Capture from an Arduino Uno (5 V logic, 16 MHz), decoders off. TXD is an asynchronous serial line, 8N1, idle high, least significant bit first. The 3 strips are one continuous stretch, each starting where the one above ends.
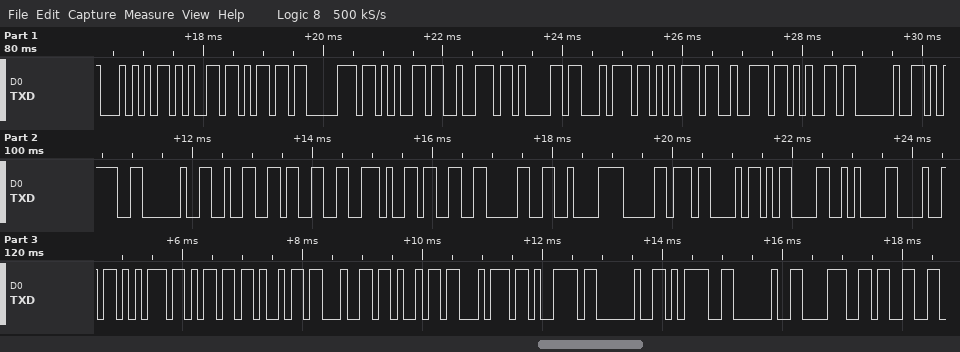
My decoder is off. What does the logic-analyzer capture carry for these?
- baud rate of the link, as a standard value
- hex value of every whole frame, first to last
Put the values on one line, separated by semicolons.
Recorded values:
9600 baud; 0x54 0x65 0x6D 0x70 0x65 0x72 0x61 0x74 0x75 0x72 0x65 0x20 0x3D 0x20 0x32 0x33 0x2E 0x33 0x30 0xC2 0xB0 0x43 0x0D 0x0A 0x48 0x75 0x6D 0x69 0x64 0x69 0x74 0x79 0x20 0x3D 0x20 0x38 0x33
